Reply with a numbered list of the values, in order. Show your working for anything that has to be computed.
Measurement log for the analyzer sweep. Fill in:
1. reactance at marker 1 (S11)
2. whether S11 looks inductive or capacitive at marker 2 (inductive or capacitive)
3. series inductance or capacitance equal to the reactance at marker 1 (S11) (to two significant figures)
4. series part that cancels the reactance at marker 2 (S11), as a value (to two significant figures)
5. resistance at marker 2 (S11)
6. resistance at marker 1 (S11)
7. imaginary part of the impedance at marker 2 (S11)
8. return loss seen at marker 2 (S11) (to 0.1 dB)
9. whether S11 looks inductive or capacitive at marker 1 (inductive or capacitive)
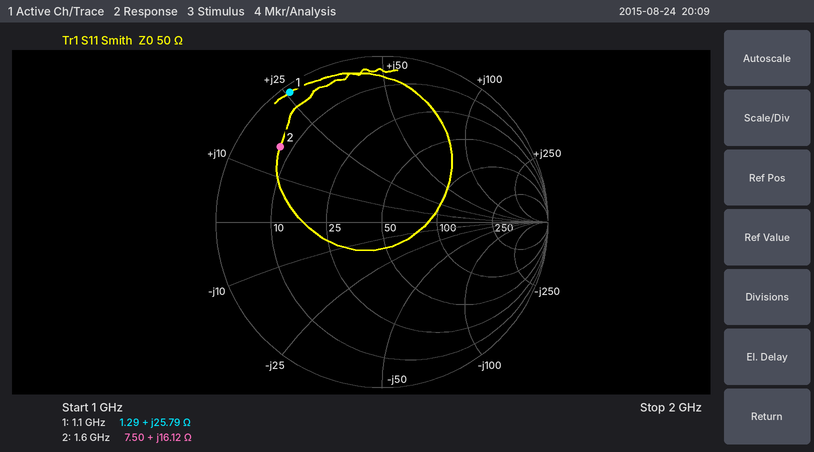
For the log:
1. +25.79 Ω
2. inductive
3. L = 25.79 Ω/(2π × 1.1 GHz) ≈ 3.7 nH
4. C = 1/(2π × 1.6 GHz × 16.12 Ω) ≈ 6.2 pF
5. 7.50 Ω
6. 1.29 Ω
7. +16.12 Ω
8. 2.4 dB
9. inductive
